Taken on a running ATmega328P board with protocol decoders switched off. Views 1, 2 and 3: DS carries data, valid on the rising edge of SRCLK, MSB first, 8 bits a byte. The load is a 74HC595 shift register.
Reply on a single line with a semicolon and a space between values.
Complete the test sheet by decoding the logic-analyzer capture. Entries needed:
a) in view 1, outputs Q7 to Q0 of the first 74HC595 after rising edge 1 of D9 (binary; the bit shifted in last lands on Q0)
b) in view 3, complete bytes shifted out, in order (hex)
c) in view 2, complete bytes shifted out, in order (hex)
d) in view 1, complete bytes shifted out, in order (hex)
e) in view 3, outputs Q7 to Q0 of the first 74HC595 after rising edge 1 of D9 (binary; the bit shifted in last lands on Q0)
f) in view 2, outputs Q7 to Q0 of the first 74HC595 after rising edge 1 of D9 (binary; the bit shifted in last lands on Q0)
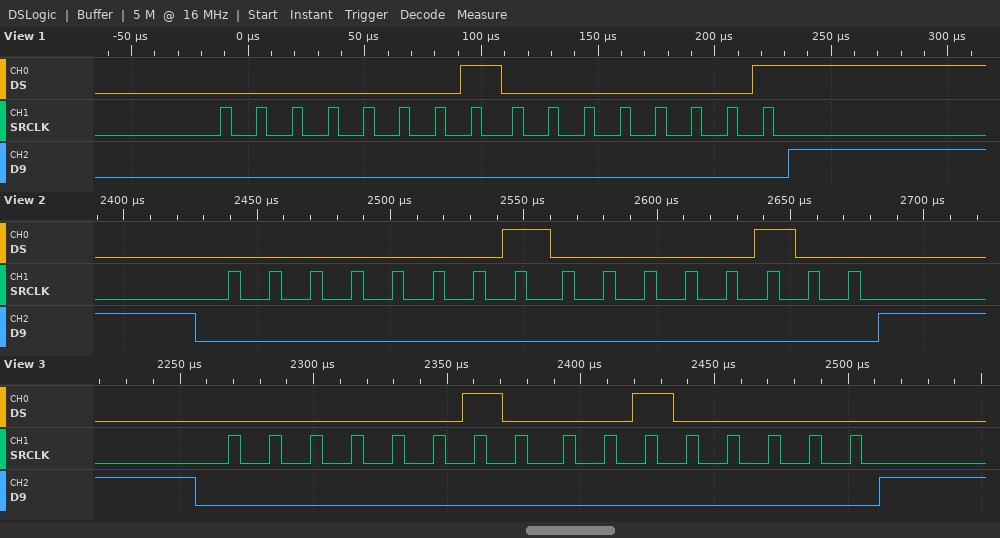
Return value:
00000001; 0x02 0x20; 01 04; 0x01 0x01; 00100000; 00000100
